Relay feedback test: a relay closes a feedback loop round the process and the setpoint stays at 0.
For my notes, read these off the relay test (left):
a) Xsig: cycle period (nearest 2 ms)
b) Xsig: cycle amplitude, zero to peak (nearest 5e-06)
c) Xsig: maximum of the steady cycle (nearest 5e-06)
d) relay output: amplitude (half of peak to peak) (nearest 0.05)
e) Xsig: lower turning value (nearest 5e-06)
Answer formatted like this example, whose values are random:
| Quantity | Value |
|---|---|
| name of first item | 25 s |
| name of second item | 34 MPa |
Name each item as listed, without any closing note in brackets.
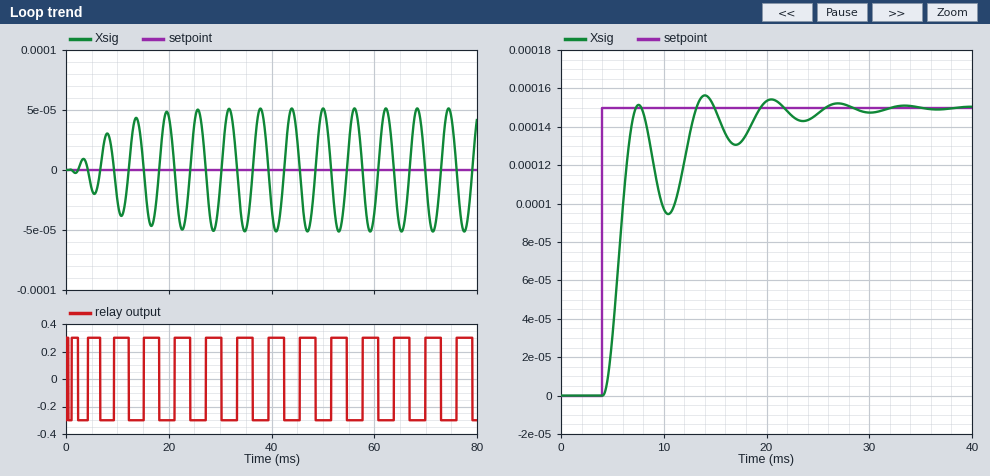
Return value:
| Quantity | Value |
|---|---|
| Xsig: cycle period | 6 ms |
| Xsig: cycle amplitude, zero to peak | 0.000050 |
| Xsig: maximum of the steady cycle | 0.000050 |
| relay output: amplitude (half of peak to peak) | 0.30 |
| Xsig: lower turning value | -0.000050 |
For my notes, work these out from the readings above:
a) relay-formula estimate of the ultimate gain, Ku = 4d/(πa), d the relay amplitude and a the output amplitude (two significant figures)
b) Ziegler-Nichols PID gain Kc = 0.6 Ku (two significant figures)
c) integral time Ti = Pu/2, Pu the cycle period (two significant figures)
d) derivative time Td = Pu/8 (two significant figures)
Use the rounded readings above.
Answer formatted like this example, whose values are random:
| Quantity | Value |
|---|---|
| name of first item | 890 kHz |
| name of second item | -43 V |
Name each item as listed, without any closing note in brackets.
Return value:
| Quantity | Value |
|---|---|
| relay-formula estimate of the ultimate gain, Ku = 4d/(πa), d the relay amplitude and a the output amplitude | 7600 |
| Ziegler-Nichols PID gain Kc = 0.6 Ku | 4600 |
| integral time Ti = Pu/2, Pu the cycle period | 3.0 ms |
| derivative time Td = Pu/8 | 0.75 ms |
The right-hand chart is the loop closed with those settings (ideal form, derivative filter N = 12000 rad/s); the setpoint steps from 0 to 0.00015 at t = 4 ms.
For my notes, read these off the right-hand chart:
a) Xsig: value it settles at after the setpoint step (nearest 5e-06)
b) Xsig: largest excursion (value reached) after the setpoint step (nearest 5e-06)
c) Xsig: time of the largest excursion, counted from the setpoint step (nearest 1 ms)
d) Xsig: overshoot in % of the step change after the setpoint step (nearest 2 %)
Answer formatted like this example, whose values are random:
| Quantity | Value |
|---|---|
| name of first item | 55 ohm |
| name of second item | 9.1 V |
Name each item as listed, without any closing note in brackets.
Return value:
| Quantity | Value |
|---|---|
| Xsig: value it settles at after the setpoint step | 0.000150 |
| Xsig: largest excursion (value reached) after the setpoint step | 0.000155 |
| Xsig: time of the largest excursion, counted from the setpoint step | 10 ms |
| Xsig: overshoot in % of the step change after the setpoint step | 4 % |
